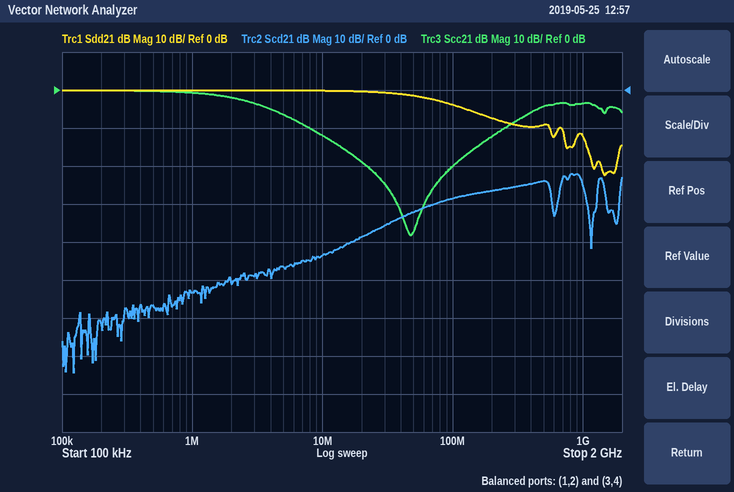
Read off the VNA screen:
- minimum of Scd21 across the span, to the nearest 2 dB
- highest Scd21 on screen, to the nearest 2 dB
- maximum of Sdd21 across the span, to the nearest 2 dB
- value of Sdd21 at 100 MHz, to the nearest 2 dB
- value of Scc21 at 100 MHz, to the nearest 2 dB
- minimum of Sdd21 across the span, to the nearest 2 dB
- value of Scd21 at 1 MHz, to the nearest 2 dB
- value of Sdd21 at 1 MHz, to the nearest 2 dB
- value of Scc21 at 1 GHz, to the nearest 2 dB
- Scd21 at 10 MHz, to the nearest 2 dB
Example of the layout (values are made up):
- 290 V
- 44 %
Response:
- -74 dB
- -22 dB
- 0 dB
- -4 dB
- -20 dB
- -22 dB
- -54 dB
- 0 dB
- -4 dB
- -44 dB
